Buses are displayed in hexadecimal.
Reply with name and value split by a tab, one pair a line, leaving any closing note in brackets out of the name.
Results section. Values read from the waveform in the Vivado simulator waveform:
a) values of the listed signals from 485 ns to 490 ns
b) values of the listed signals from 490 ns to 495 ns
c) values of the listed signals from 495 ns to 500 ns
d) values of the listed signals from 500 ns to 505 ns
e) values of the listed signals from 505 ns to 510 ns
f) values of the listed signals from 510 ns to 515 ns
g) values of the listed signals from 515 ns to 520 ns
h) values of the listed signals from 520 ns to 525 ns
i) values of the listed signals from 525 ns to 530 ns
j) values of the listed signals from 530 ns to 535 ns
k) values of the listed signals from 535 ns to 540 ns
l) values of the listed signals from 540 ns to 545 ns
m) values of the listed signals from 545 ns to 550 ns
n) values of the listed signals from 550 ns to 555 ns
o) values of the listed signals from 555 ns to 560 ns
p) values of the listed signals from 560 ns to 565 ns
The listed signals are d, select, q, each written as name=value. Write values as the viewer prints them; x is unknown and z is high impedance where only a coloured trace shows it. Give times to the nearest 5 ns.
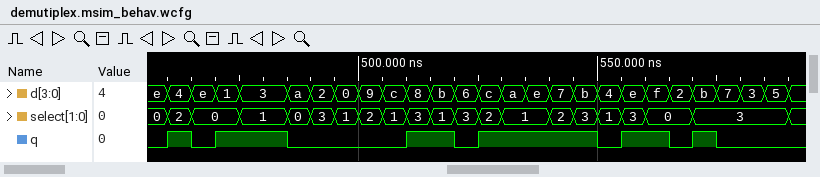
values of the listed signals from 485 ns to 490 ns	d=a, select=0, q=0
values of the listed signals from 490 ns to 495 ns	d=2, select=3, q=0
values of the listed signals from 495 ns to 500 ns	d=0, select=1, q=0
values of the listed signals from 500 ns to 505 ns	d=9, select=2, q=0
values of the listed signals from 505 ns to 510 ns	d=c, select=1, q=0
values of the listed signals from 510 ns to 515 ns	d=8, select=3, q=1
values of the listed signals from 515 ns to 520 ns	d=b, select=1, q=1
values of the listed signals from 520 ns to 525 ns	d=6, select=3, q=0
values of the listed signals from 525 ns to 530 ns	d=c, select=2, q=1
values of the listed signals from 530 ns to 535 ns	d=a, select=1, q=1
values of the listed signals from 535 ns to 540 ns	d=e, select=1, q=1
values of the listed signals from 540 ns to 545 ns	d=7, select=2, q=1
values of the listed signals from 545 ns to 550 ns	d=b, select=3, q=1
values of the listed signals from 550 ns to 555 ns	d=4, select=1, q=0
values of the listed signals from 555 ns to 560 ns	d=e, select=3, q=1
values of the listed signals from 560 ns to 565 ns	d=f, select=0, q=1
